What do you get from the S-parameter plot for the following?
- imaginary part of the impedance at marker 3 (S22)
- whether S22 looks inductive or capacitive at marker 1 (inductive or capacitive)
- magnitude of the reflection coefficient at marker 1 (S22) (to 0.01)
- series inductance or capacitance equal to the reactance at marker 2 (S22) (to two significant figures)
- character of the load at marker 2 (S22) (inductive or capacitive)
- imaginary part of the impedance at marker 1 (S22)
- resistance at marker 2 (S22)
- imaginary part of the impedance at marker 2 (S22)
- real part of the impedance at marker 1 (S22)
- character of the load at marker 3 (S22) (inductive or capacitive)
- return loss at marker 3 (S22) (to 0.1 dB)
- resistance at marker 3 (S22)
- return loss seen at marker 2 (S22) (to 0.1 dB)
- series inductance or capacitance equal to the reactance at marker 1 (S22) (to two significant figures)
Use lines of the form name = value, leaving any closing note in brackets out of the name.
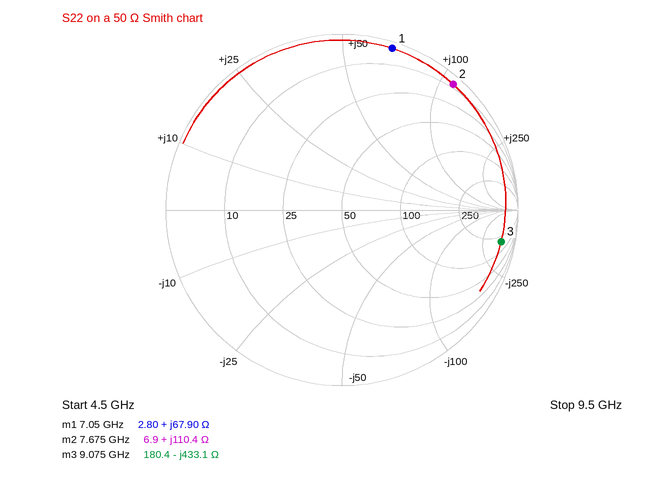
imaginary part of the impedance at marker 3 = -433.1 Ω
whether S22 looks inductive or capacitive at marker 1 = inductive
magnitude of the reflection coefficient at marker 1 (S22) = 0.96
series inductance or capacitance equal to the reactance at marker 2 (S22) = 2.3 nH
character of the load at marker 2 (S22) = inductive
imaginary part of the impedance at marker 1 = +67.90 Ω
resistance at marker 2 = 6.9 Ω
imaginary part of the impedance at marker 2 = +110.4 Ω
real part of the impedance at marker 1 = 2.80 Ω
character of the load at marker 3 (S22) = capacitive
return loss at marker 3 (S22) = 0.7 dB
resistance at marker 3 = 180.4 Ω
return loss seen at marker 2 (S22) = 0.4 dB
series inductance or capacitance equal to the reactance at marker 1 (S22) = 1.5 nH
